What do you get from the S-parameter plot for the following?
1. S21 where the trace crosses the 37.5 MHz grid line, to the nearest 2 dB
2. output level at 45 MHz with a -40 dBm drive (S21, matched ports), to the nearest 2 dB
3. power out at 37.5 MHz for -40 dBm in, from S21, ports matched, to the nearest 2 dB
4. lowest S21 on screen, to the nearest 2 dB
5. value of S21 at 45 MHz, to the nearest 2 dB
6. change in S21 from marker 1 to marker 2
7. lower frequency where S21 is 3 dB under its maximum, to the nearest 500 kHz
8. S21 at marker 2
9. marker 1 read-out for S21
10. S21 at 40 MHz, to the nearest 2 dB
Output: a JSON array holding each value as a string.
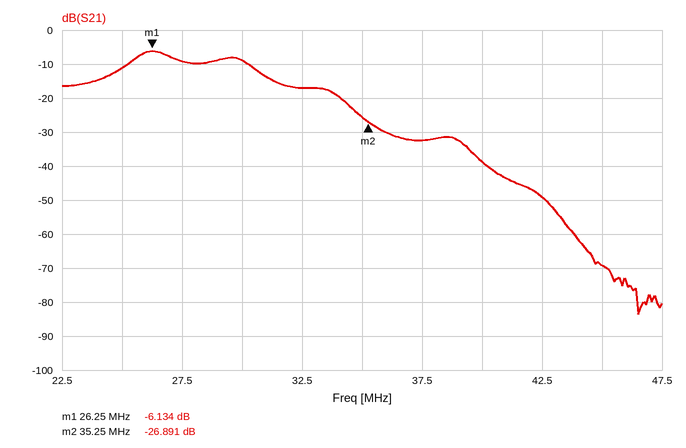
["-32 dB", "-110 dBm", "-72 dBm", "-84 dB", "-70 dB", "-20.757 dB", "25.5 MHz", "-26.891 dB", "-6.134 dB", "-38 dB"]
